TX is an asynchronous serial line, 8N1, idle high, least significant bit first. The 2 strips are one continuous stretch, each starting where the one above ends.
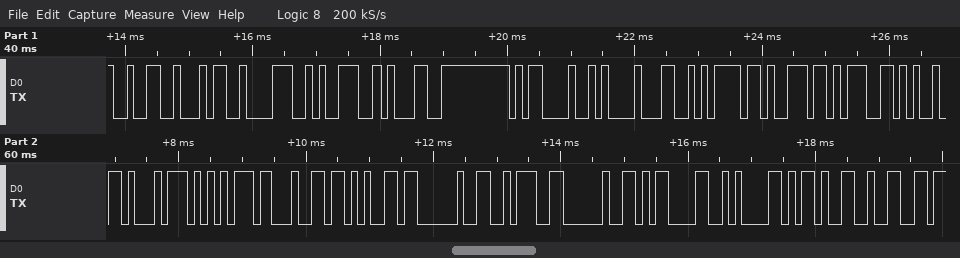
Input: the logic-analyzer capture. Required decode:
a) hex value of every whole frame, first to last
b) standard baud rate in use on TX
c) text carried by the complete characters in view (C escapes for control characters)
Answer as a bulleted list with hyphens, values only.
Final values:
- 32 34 38 39 31 0D 0A 4C 6F 6E 67 69 74 75 64 65 20 3A 20 0D 0A 2D 32
- 9600 baud
- "24891\r\nLongitude : \r\n-2"
